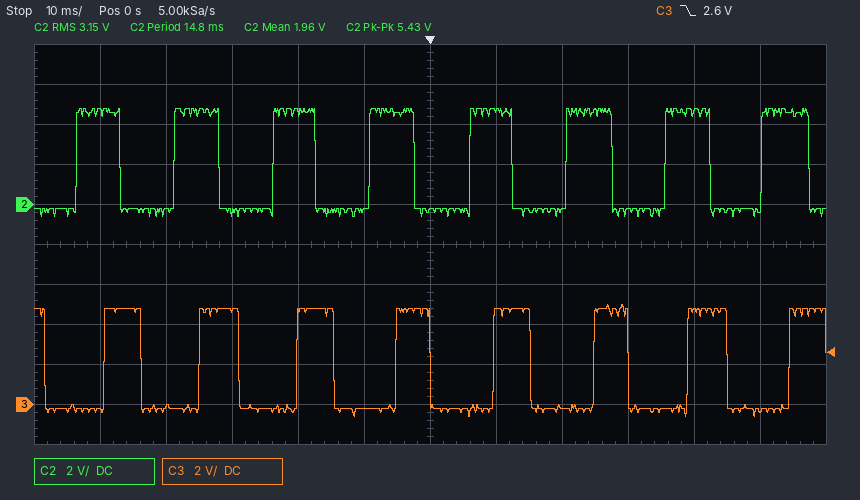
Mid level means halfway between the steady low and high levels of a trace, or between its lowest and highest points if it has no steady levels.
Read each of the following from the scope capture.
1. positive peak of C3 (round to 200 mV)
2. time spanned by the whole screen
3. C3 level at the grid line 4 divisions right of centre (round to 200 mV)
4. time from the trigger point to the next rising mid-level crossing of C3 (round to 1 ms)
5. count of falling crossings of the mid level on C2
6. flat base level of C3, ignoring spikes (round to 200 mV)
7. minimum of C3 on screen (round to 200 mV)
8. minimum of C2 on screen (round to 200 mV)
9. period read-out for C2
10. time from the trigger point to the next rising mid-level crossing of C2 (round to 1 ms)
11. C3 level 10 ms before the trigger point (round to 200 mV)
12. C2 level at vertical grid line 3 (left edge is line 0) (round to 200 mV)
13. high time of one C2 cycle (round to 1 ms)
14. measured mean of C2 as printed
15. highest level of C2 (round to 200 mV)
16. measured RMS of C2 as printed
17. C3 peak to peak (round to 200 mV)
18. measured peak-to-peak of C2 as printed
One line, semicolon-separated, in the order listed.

5.0 V; 120 ms; 4.8 V; 10 ms; 8; -200 mV; -600 mV; -600 mV; 14.8 ms; 6 ms; -200 mV; -400 mV; 7 ms; 1.96 V; 4.8 V; 3.15 V; 5.6 V; 5.43 V
